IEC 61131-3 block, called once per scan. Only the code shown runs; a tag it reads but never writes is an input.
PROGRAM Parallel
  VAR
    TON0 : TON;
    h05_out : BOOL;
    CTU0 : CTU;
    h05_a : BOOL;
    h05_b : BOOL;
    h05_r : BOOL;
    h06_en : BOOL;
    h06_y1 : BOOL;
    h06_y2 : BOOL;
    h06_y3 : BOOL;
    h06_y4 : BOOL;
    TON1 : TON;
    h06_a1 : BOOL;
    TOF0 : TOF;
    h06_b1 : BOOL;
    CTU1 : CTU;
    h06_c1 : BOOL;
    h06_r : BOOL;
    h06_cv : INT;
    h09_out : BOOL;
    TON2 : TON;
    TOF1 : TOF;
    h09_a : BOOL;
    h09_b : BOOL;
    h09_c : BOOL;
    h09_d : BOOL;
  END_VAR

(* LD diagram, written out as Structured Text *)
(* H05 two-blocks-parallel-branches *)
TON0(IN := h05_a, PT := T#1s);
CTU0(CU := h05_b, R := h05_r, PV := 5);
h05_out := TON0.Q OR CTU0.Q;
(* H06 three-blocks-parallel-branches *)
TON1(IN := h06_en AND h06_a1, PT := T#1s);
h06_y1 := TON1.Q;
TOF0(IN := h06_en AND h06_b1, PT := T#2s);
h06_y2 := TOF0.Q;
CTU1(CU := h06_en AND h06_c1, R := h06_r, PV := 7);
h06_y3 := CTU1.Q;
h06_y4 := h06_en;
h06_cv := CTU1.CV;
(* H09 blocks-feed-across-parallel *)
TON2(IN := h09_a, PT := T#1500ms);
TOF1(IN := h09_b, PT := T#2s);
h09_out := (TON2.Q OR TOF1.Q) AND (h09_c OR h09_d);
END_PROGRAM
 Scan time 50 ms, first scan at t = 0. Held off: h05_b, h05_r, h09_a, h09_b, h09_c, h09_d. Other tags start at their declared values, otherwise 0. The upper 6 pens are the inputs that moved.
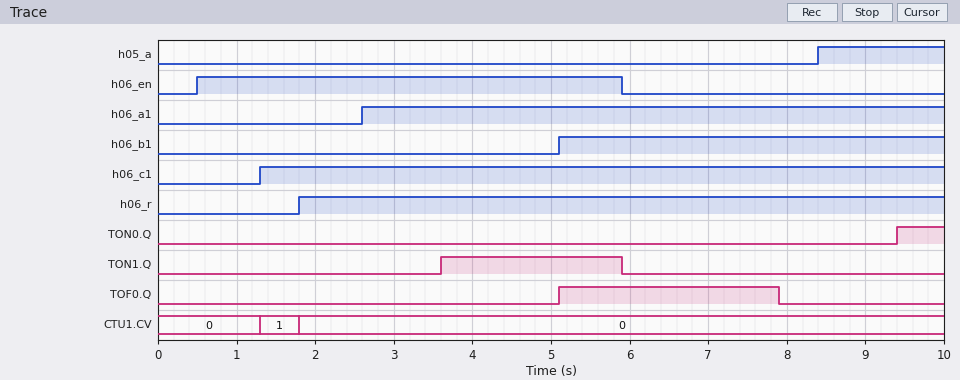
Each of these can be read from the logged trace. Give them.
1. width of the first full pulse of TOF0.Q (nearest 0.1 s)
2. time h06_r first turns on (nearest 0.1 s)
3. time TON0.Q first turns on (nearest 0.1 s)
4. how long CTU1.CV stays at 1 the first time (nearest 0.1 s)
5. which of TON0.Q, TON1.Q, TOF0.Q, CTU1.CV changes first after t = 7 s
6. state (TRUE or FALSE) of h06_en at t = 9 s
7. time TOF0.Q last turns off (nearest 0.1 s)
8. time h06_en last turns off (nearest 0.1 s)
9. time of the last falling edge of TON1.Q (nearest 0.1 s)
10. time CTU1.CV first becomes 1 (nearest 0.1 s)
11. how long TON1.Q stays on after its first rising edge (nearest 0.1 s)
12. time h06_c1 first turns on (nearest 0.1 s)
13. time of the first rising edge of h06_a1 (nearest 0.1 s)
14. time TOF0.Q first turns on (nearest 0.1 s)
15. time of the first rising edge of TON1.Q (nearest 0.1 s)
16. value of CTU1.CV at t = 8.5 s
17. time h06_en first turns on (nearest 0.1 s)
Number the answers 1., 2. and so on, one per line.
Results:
1. 2.8 s
2. 1.8 s
3. 9.4 s
4. 0.5 s
5. TOF0.Q
6. FALSE
7. 7.9 s
8. 5.9 s
9. 5.9 s
10. 1.3 s
11. 2.3 s
12. 1.3 s
13. 2.6 s
14. 5.1 s
15. 3.6 s
16. 0
17. 0.5 s
